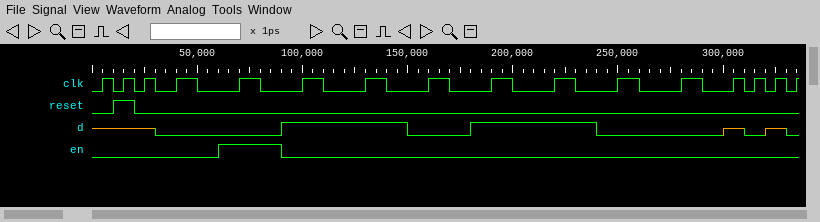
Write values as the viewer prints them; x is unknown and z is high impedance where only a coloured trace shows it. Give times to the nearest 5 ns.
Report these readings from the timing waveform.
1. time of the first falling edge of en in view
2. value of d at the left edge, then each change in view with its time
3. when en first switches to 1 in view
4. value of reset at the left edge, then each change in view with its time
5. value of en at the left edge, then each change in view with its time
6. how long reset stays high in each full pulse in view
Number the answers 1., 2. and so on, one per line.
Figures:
1. 90 ns
2. z, 0 at 30 ns, 1 at 90 ns, 0 at 150 ns, 1 at 180 ns, 0 at 240 ns, z at 300 ns, 0 at 310 ns, z at 320 ns, 0 at 330 ns
3. 60 ns
4. 0, 1 at 10 ns, 0 at 20 ns
5. 0, 1 at 60 ns, 0 at 90 ns
6. 10 ns
